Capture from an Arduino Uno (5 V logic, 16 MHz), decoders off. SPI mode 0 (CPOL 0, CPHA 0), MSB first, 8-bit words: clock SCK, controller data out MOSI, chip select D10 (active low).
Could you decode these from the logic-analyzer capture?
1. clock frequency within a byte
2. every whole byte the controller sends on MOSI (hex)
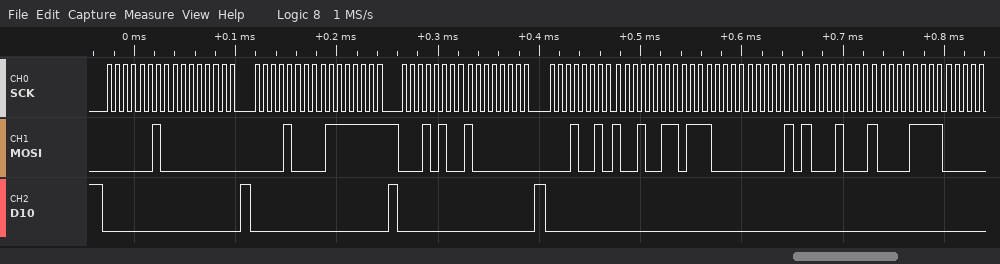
125 kHz
02 00 08 7F 14 80 12 93 70 05 11 0F
